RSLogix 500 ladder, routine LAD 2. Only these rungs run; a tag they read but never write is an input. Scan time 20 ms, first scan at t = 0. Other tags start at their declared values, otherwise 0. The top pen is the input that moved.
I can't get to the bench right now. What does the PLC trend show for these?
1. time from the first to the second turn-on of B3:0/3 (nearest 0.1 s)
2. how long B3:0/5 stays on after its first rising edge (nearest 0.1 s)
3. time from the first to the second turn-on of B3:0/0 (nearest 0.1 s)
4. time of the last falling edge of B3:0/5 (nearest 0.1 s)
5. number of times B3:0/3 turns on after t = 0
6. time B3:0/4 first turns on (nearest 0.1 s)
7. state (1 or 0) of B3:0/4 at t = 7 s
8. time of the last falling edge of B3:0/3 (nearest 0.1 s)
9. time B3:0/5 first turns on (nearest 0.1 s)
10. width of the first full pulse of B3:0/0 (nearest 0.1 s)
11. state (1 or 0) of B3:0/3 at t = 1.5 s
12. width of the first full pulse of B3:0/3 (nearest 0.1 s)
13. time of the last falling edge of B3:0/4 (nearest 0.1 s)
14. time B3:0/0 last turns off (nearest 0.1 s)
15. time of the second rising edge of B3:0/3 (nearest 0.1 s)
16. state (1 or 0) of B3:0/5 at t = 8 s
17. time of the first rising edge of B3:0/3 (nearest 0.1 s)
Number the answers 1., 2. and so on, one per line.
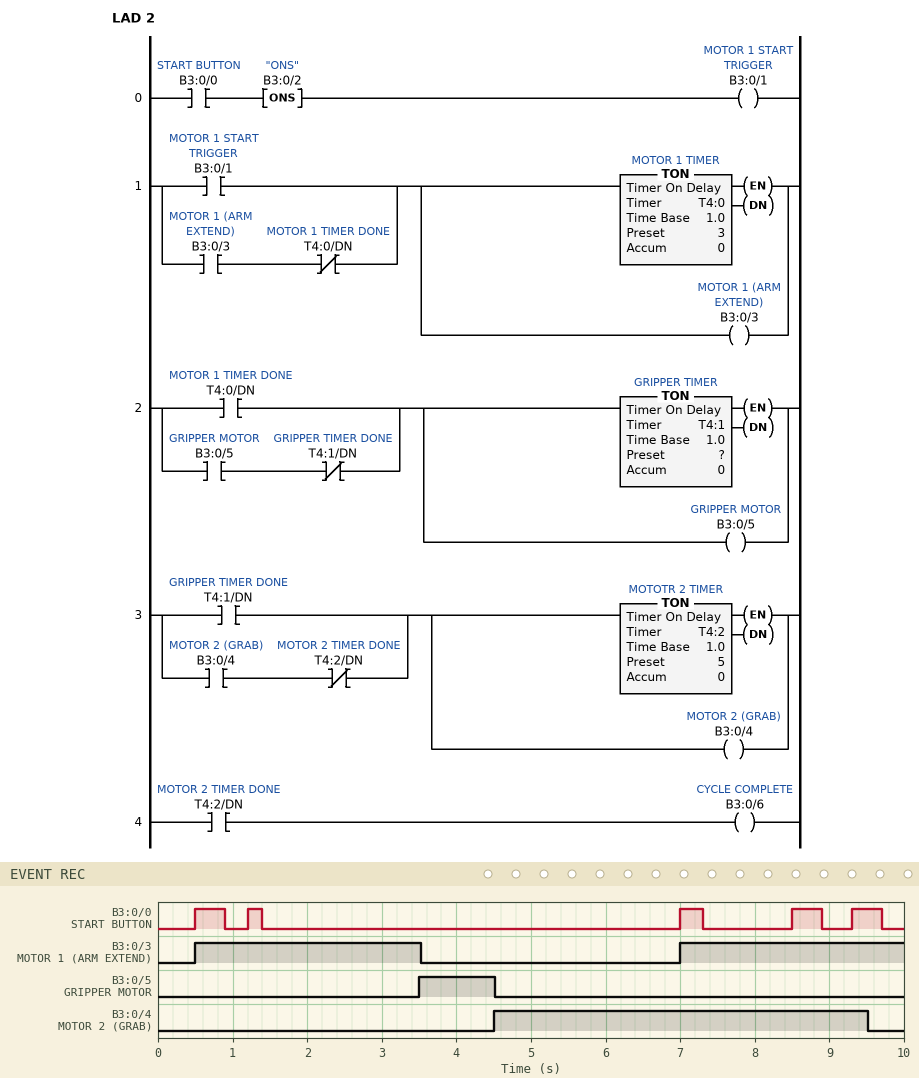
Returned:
1. 6.5 s
2. 1.0 s
3. 0.7 s
4. 4.5 s
5. 2
6. 4.5 s
7. 1
8. 3.5 s
9. 3.5 s
10. 0.4 s
11. 1
12. 3.0 s
13. 9.5 s
14. 9.7 s
15. 7.0 s
16. 0
17. 0.5 s
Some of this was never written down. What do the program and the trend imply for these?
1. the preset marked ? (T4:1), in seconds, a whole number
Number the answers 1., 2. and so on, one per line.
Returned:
1. 1 s
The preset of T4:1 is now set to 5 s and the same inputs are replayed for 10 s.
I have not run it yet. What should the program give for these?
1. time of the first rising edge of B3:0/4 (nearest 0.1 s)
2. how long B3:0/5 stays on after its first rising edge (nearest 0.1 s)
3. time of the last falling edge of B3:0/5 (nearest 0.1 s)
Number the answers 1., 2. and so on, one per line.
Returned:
1. 8.5 s
2. 5.0 s
3. 8.5 s
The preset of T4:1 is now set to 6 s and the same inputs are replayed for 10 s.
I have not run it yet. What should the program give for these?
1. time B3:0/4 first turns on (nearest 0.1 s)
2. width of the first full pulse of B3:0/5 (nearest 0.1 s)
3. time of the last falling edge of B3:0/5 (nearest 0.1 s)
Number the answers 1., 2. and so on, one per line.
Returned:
1. 9.5 s
2. 6.0 s
3. 9.5 s
